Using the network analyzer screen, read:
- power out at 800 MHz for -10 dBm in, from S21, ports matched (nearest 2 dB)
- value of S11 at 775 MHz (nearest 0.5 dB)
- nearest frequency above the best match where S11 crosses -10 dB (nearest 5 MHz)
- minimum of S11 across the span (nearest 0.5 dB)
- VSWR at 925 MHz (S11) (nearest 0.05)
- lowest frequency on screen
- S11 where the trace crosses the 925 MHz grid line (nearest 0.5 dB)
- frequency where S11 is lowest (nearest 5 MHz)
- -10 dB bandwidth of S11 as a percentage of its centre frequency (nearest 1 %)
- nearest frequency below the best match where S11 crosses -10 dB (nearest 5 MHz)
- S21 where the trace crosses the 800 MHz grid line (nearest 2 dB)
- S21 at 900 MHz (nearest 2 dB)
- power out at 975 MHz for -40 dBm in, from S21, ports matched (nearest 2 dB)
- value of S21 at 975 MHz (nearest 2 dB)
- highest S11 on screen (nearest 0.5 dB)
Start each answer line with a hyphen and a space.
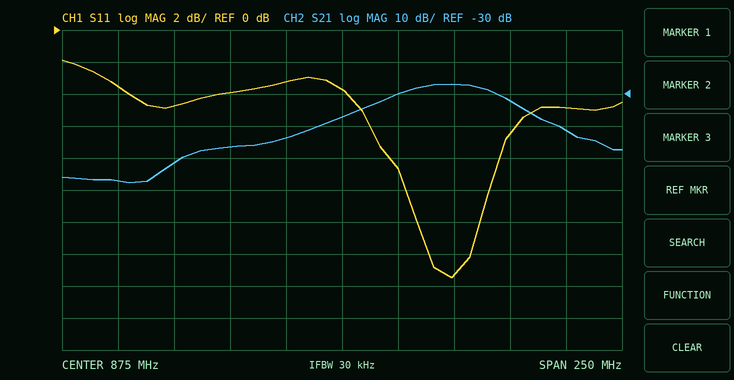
- -62 dBm
- -3.5 dB
- 940 MHz
- -15.5 dB
- 1.40
- 750 MHz
- -15.5 dB
- 925 MHz
- 4 %
- 905 MHz
- -52 dB
- -30 dB
- -82 dBm
- -42 dB
- -2.0 dB
